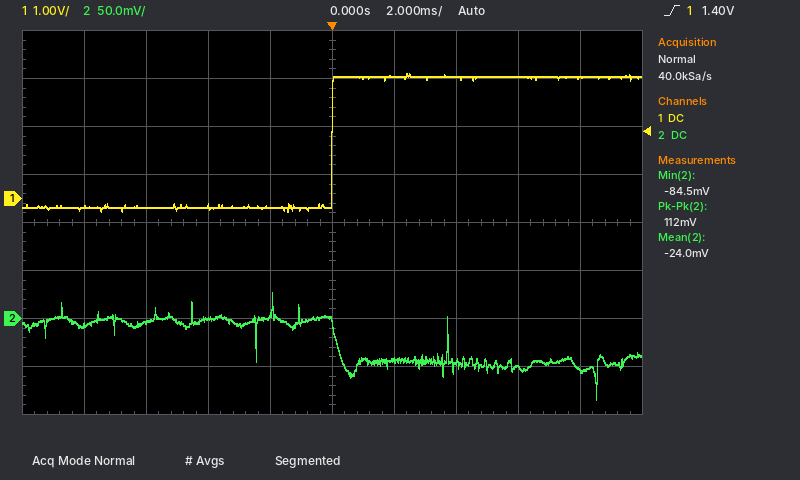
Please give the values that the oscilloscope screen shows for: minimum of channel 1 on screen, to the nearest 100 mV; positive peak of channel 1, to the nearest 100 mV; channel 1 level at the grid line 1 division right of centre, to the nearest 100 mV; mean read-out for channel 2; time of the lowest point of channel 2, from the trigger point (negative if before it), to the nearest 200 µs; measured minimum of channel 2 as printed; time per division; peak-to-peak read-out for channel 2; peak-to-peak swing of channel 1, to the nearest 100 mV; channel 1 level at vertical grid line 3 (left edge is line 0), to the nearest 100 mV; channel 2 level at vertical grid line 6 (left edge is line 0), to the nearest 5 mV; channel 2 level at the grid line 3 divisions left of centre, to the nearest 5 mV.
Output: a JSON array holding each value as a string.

["-300 mV", "2.6 V", "2.5 V", "-24.0 mV", "+8.6 ms", "-84.5 mV", "2 ms", "112 mV", "2.9 V", "-200 mV", "-45 mV", "-5 mV"]
